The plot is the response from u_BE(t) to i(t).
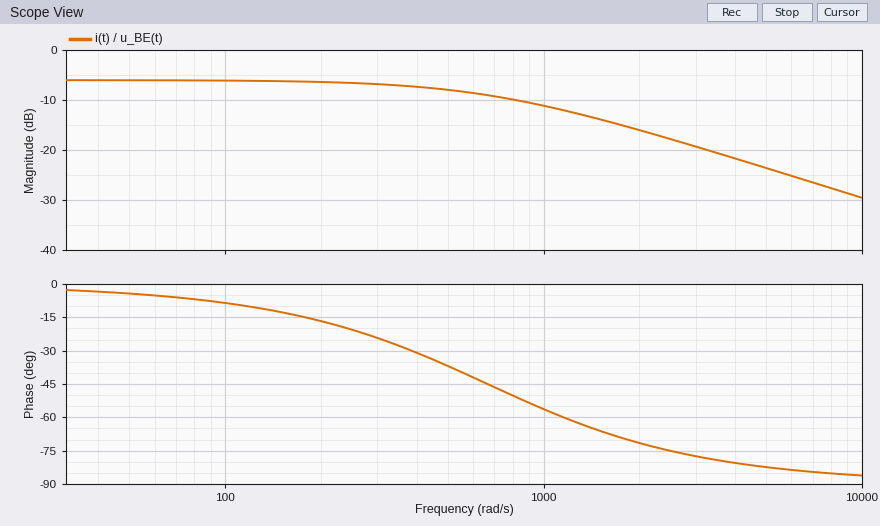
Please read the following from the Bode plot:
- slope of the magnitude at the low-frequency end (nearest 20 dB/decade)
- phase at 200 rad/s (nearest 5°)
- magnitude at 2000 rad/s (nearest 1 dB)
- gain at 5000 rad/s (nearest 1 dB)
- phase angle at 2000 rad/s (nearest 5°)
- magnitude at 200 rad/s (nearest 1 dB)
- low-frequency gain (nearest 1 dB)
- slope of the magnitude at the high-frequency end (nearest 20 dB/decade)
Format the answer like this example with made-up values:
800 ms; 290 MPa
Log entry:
0 dB/decade; -15°; -16 dB; -24 dB; -70°; -6 dB; -6 dB; -20 dB/decade
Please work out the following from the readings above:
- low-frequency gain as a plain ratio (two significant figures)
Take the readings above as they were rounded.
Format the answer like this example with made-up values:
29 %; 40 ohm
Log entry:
0.50
